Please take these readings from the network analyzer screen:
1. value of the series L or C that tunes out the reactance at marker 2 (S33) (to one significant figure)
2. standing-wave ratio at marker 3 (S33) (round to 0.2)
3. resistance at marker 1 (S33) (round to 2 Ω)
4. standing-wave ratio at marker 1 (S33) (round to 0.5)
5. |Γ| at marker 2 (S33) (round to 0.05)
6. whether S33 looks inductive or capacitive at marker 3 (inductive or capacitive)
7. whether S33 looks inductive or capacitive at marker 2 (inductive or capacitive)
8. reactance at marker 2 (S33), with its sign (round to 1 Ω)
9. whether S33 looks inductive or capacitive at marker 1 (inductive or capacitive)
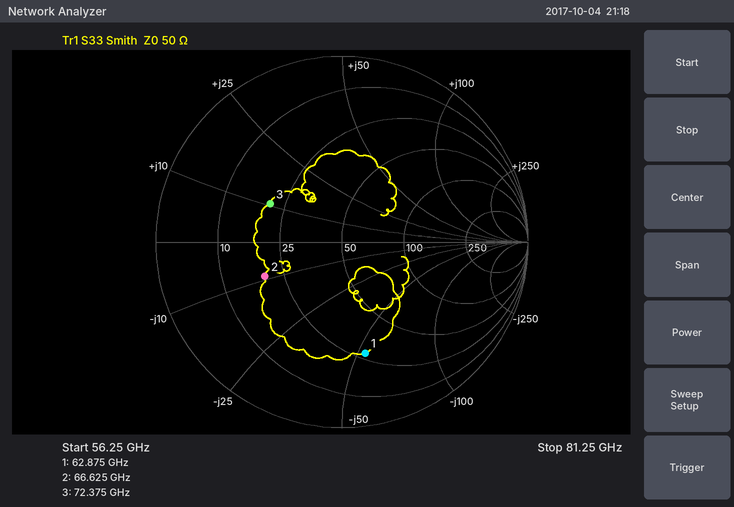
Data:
20 pH
2.6
28 Ω
4.0
0.45
inductive
capacitive
-9 Ω
capacitive
